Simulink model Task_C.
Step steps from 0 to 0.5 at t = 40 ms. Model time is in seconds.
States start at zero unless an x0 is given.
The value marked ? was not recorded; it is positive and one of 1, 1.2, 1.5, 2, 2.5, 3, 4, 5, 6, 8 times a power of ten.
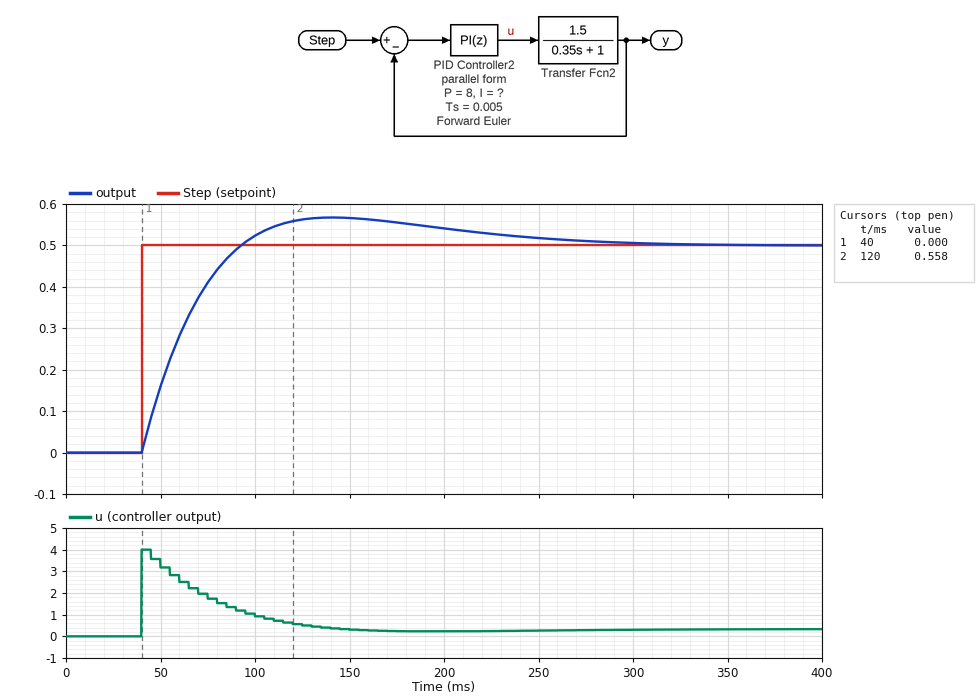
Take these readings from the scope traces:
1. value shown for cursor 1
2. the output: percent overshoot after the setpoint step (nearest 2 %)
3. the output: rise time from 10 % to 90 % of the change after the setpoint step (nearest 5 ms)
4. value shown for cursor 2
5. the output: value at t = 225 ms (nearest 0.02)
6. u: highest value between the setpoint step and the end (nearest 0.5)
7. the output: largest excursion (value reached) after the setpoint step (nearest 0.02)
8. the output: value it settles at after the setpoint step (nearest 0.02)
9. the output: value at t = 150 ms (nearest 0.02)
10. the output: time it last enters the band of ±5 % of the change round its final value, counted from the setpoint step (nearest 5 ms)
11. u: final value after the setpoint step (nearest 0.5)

0.000
14 %
40 ms
0.558
0.52
4.0
0.56
0.50
0.56
190 ms
0.5
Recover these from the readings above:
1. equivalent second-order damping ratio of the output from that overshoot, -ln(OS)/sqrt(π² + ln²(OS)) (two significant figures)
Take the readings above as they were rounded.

0.53
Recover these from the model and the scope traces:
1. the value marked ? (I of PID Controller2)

100
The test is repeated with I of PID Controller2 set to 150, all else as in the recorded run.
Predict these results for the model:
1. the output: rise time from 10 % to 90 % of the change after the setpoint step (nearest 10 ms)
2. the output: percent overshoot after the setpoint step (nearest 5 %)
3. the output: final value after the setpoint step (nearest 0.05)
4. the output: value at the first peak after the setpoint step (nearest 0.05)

30 ms
20 %
0.50
0.60
